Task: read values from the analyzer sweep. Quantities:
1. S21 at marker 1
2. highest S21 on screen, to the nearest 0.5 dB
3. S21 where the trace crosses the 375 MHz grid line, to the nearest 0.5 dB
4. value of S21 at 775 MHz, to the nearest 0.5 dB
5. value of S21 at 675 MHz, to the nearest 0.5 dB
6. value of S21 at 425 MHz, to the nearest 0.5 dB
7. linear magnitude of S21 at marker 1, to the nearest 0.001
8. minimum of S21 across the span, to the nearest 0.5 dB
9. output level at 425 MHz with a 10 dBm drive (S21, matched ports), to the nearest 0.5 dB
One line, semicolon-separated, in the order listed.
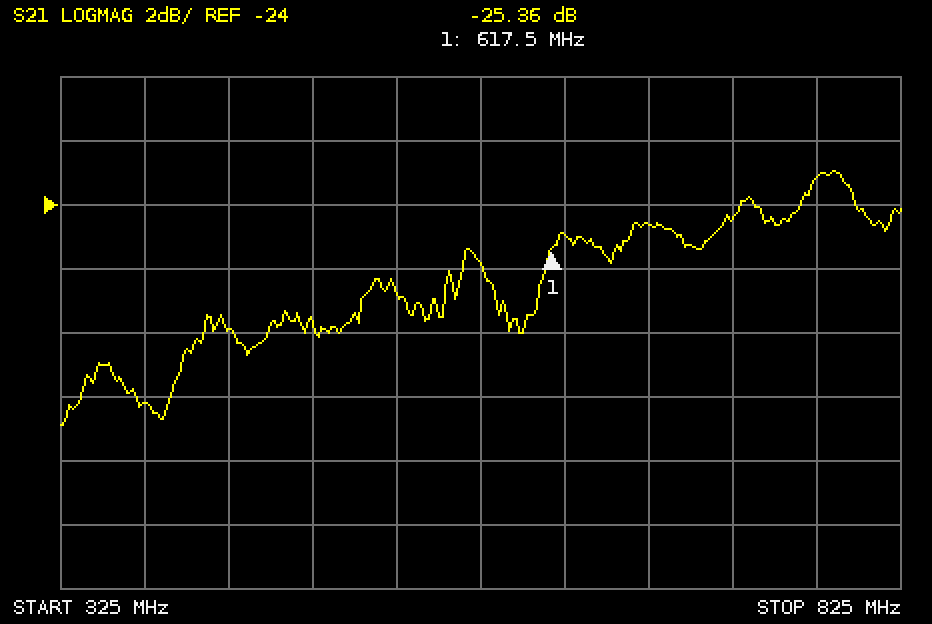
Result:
-25.36 dB; -23.0 dB; -30.0 dB; -23.0 dB; -24.5 dB; -28.0 dB; 0.054; -31.0 dB; -18.0 dBm
